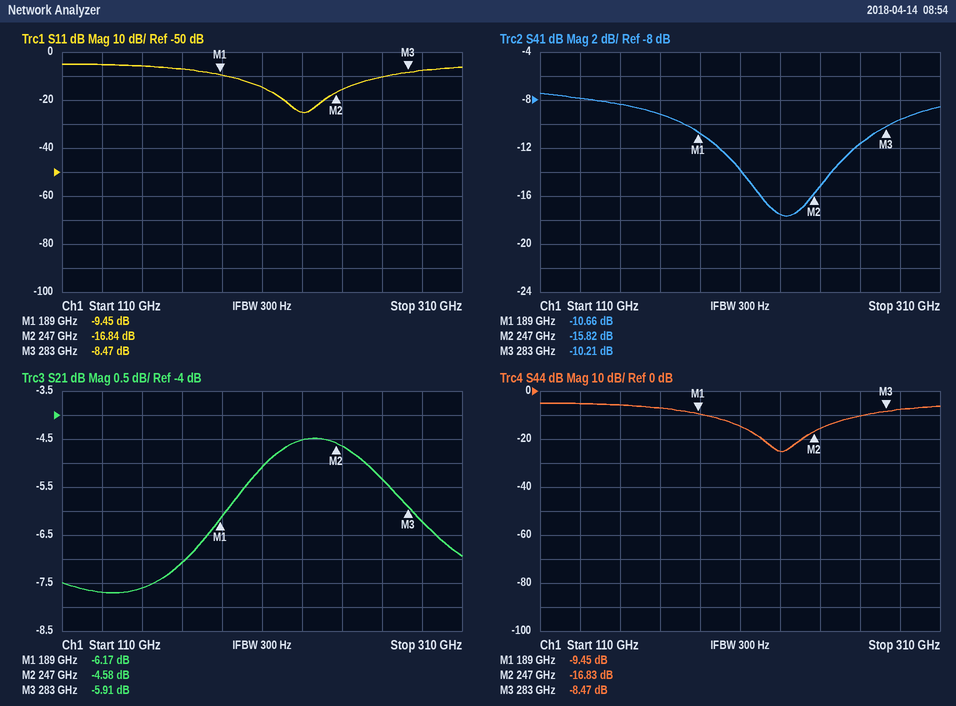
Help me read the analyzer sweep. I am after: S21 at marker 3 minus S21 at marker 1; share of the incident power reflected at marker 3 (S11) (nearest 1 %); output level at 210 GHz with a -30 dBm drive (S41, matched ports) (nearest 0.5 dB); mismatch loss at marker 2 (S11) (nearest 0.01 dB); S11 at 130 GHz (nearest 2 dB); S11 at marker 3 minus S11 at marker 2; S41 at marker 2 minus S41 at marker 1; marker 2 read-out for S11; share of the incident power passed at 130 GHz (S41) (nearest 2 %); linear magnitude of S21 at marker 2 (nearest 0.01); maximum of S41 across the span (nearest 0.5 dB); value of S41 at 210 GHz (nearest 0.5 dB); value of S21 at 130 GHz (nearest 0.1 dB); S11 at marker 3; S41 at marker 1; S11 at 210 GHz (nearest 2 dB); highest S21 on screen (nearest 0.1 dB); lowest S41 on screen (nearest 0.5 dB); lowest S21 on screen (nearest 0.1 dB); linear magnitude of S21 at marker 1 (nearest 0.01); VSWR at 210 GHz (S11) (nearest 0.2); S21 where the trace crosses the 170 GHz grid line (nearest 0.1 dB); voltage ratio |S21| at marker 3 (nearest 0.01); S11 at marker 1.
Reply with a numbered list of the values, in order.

1. 0.26 dB
2. 14 %
3. -44.0 dBm
4. 0.09 dB
5. -6 dB
6. 8.37 dB
7. -5.16 dB
8. -16.84 dB
9. 16 %
10. 0.59
11. -7.5 dB
12. -14.0 dB
13. -7.7 dB
14. -8.47 dB
15. -10.66 dB
16. -14 dB
17. -4.5 dB
18. -17.5 dB
19. -7.7 dB
20. 0.49
21. 1.4
22. -7.1 dB
23. 0.51
24. -9.45 dB
